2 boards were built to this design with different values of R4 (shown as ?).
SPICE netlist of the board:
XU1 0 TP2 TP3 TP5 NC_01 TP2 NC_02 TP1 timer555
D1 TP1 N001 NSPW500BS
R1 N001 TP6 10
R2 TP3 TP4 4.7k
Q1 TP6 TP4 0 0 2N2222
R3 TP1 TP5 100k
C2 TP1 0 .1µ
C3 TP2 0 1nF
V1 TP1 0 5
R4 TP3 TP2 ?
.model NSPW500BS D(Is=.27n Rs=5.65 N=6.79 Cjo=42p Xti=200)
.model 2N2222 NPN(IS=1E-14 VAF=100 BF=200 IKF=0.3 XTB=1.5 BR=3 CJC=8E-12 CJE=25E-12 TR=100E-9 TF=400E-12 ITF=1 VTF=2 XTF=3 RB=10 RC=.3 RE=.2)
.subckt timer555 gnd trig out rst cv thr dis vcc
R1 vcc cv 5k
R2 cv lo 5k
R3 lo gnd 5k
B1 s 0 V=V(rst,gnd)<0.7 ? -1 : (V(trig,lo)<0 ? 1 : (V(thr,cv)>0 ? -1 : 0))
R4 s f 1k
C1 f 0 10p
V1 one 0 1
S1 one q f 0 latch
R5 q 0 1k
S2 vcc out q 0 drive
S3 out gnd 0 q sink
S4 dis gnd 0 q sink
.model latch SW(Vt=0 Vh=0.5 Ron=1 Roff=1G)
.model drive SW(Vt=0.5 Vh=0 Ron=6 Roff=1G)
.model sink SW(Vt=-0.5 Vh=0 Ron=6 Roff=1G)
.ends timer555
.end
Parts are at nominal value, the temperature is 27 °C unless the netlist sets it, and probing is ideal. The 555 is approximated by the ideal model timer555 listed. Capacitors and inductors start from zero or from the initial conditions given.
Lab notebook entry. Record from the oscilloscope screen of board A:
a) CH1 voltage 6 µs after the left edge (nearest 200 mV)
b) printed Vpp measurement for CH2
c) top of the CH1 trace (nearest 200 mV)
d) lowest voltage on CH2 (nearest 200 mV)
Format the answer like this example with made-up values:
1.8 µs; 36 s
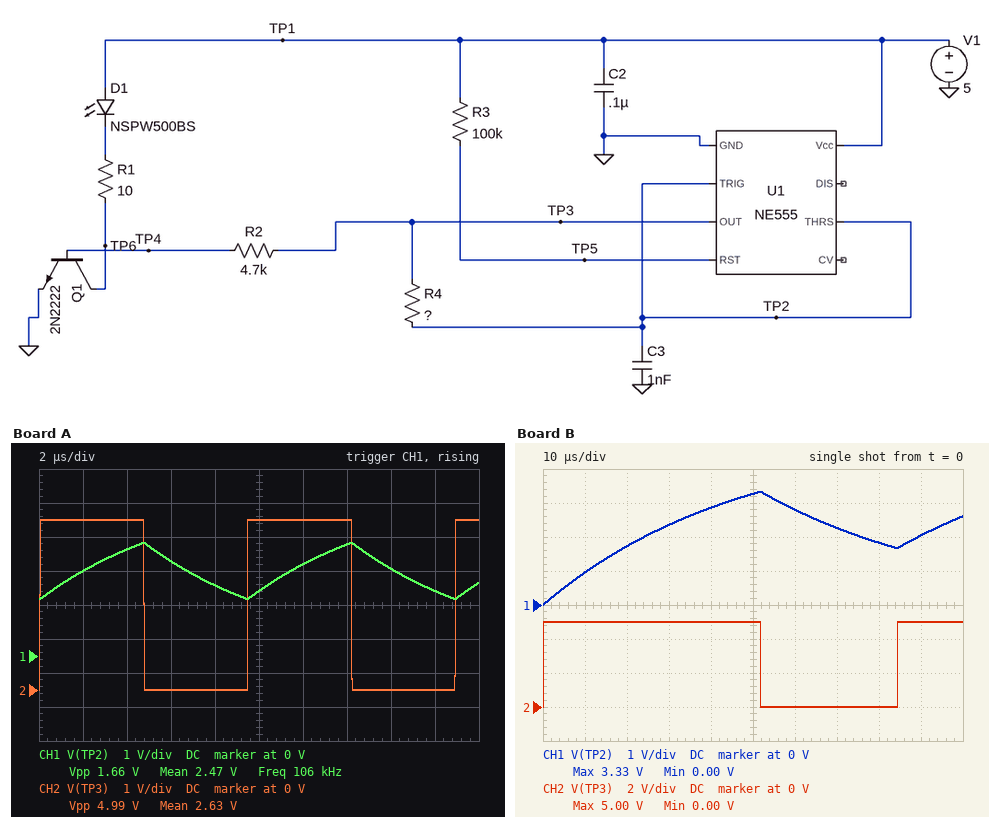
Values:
2.8 V; 4.99 V; 3.4 V; 0 V
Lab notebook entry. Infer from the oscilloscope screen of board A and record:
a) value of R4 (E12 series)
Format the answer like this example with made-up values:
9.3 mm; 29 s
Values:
6.8 kΩ
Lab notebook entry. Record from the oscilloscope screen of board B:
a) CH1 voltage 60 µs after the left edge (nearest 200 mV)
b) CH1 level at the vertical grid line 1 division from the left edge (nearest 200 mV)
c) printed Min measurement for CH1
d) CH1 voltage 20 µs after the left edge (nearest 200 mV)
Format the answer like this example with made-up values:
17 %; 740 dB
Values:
2.8 V; 1.0 V; 0.00 V; 1.8 V
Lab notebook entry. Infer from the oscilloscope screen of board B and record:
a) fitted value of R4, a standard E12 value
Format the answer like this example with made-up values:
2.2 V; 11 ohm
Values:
47 kΩ
